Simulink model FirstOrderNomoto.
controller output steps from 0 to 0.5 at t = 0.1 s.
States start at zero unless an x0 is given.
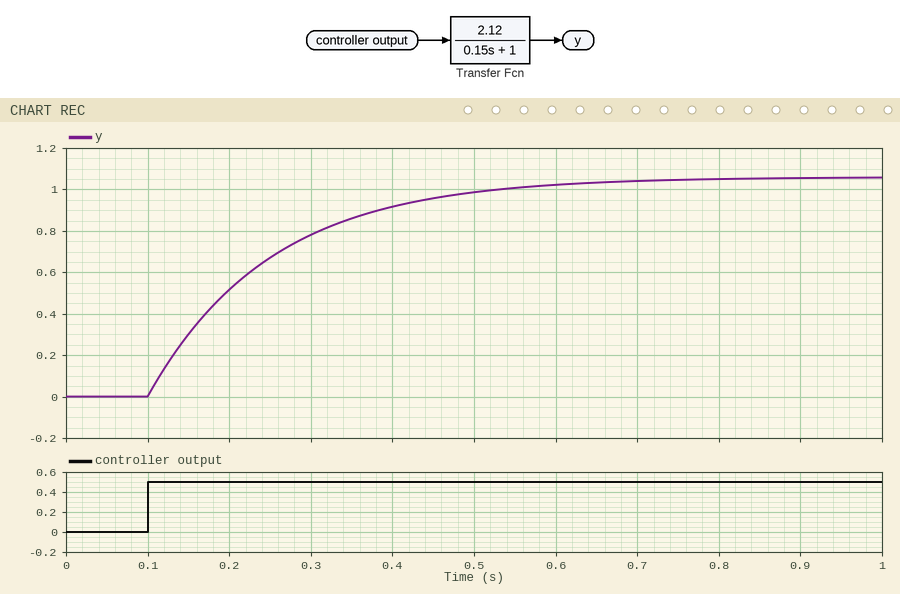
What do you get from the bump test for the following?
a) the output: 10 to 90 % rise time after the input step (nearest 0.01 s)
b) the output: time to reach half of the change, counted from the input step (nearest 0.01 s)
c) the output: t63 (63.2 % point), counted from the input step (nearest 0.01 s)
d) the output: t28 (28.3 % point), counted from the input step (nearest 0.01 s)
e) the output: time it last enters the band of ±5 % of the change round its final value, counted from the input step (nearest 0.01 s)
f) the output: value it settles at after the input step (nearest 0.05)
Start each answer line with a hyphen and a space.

- 0.33 s
- 0.10 s
- 0.15 s
- 0.05 s
- 0.45 s
- 1.05
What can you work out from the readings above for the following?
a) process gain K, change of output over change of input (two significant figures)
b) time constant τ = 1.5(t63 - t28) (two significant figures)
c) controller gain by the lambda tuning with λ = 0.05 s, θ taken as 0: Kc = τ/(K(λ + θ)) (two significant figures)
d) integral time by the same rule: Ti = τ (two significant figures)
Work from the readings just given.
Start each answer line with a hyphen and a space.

- 2.1
- 0.15 s
- 1.4
- 0.15 s
